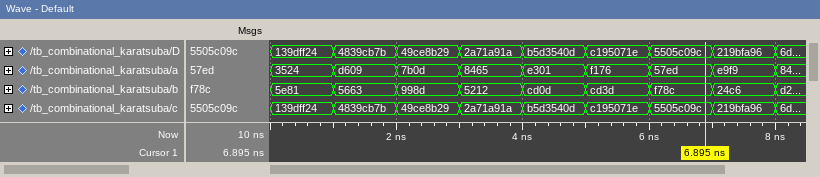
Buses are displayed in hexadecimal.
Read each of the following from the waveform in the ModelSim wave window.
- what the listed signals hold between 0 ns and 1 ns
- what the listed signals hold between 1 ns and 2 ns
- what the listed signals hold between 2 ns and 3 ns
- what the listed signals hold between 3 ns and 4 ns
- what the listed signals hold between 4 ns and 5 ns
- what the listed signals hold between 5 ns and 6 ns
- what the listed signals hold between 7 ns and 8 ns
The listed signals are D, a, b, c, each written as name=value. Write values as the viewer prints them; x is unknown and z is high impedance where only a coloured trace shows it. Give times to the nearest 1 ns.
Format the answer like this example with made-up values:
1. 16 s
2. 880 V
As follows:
1. D=139dff24, a=3524, b=5e81, c=139dff24
2. D=4839cb7b, a=d609, b=5663, c=4839cb7b
3. D=49ce8b29, a=7b0d, b=998d, c=49ce8b29
4. D=2a71a91a, a=8465, b=5212, c=2a71a91a
5. D=b5d3540d, a=e301, b=cd0d, c=b5d3540d
6. D=c195071e, a=f176, b=cd3d, c=c195071e
7. D=219bfa96, a=e9f9, b=24c6, c=219bfa96
